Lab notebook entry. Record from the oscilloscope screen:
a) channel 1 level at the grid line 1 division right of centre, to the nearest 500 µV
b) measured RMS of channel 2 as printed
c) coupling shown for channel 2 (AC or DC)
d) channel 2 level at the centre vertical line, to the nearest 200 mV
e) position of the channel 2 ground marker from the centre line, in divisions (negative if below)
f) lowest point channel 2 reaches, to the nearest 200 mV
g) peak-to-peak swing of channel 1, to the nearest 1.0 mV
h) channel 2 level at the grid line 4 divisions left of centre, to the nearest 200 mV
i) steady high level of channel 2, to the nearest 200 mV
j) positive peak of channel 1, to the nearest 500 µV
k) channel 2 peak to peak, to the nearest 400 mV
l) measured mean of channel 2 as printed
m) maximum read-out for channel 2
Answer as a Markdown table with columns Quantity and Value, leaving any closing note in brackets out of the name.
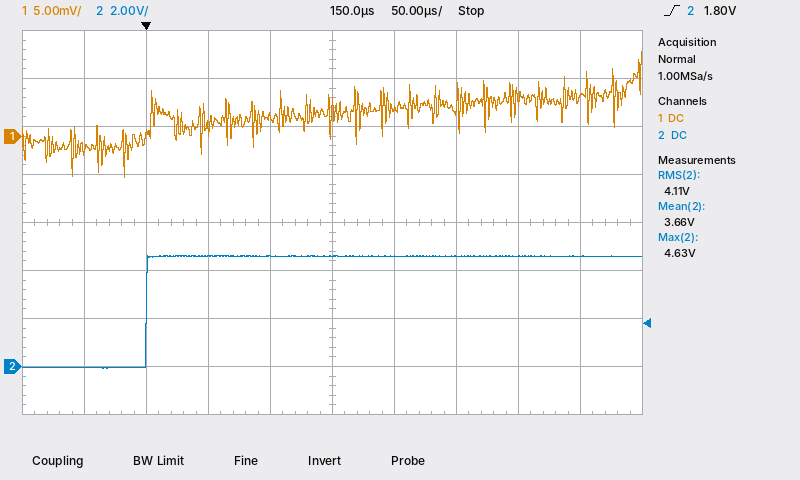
| Quantity | Value |
|---|---|
| channel 1 level at the grid line 1 division right of centre, to the nearest 500 µV | 3.0 mV |
| measured RMS of channel 2 as printed | 4.11 V |
| coupling shown for channel 2 | DC |
| channel 2 level at the centre vertical line, to the nearest 200 mV | 4.6 V |
| position of the channel 2 ground marker from the centre line, in divisions | -3.0 div |
| lowest point channel 2 reaches, to the nearest 200 mV | 0.0 V |
| peak-to-peak swing of channel 1, to the nearest 1.0 mV | 13.0 mV |
| channel 2 level at the grid line 4 divisions left of centre, to the nearest 200 mV | 0.0 V |
| steady high level of channel 2, to the nearest 200 mV | 4.6 V |
| positive peak of channel 1, to the nearest 500 µV | 9.0 mV |
| channel 2 peak to peak, to the nearest 400 mV | 4.8 V |
| measured mean of channel 2 as printed | 3.66 V |
| maximum read-out for channel 2 | 4.63 V |
